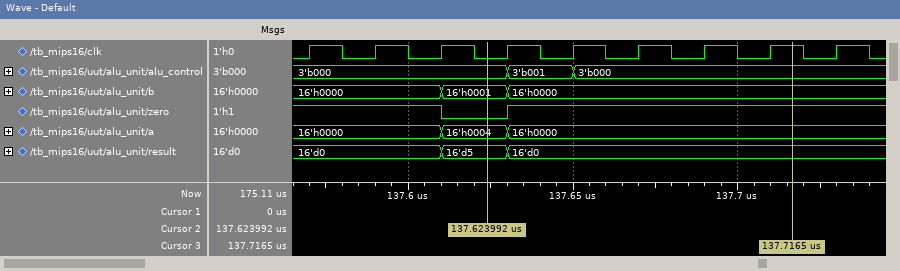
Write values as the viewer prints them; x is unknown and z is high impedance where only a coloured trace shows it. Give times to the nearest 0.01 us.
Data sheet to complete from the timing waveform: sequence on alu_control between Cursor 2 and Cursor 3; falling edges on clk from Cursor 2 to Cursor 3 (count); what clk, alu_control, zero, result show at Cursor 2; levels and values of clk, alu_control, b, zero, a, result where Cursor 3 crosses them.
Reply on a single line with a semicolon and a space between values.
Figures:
3'b000, 3'b001, 3'b000; 4; clk=0, alu_control=3'b000, zero=0, result=16'd5; clk=1, alu_control=3'b000, b=16'h0000, zero=1, a=16'h0000, result=16'd0
